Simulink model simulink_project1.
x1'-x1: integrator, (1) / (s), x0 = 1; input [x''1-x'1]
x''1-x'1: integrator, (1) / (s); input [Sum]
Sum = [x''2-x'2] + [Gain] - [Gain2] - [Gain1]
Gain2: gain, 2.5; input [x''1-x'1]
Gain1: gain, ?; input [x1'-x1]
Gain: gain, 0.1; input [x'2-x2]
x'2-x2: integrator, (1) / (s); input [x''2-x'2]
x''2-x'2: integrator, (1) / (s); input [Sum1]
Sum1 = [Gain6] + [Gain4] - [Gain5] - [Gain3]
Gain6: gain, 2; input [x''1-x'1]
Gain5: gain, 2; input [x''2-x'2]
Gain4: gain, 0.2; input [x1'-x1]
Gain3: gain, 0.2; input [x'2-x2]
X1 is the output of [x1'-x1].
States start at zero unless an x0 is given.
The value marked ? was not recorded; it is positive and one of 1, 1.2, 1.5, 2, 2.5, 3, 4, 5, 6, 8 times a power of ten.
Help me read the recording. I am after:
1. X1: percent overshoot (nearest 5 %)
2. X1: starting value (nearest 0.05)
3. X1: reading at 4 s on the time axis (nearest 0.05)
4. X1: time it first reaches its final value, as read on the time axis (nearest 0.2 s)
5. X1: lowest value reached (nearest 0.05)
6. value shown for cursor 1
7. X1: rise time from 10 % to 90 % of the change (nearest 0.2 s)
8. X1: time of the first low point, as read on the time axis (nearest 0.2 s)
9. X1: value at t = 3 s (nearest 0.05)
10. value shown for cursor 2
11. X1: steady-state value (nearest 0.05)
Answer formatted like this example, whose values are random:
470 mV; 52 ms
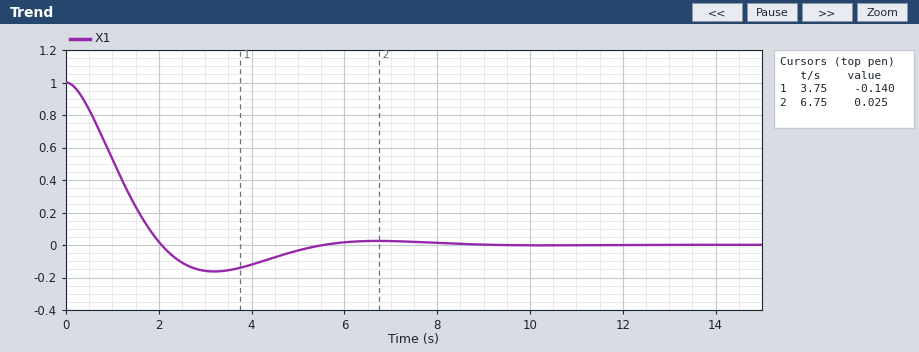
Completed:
15 %; 1.00; -0.10; 2.0 s; -0.15; -0.140; 1.4 s; 3.2 s; -0.15; 0.025; 0.00
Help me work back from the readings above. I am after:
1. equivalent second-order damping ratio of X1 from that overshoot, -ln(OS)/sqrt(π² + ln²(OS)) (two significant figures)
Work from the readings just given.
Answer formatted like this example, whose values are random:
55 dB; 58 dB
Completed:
0.52
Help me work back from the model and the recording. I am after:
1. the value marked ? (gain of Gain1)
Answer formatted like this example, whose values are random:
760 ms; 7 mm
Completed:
2
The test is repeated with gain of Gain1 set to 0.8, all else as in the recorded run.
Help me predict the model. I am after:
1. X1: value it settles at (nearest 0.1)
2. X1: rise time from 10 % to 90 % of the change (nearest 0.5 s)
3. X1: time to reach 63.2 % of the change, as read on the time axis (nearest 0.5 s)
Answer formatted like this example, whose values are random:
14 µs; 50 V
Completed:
0.0; 3.5 s; 2.5 s
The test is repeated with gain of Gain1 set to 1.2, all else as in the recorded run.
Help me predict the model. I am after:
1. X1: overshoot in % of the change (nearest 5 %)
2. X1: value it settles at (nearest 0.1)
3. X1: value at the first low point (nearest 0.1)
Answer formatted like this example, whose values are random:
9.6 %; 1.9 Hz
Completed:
10 %; 0.0; -0.1
